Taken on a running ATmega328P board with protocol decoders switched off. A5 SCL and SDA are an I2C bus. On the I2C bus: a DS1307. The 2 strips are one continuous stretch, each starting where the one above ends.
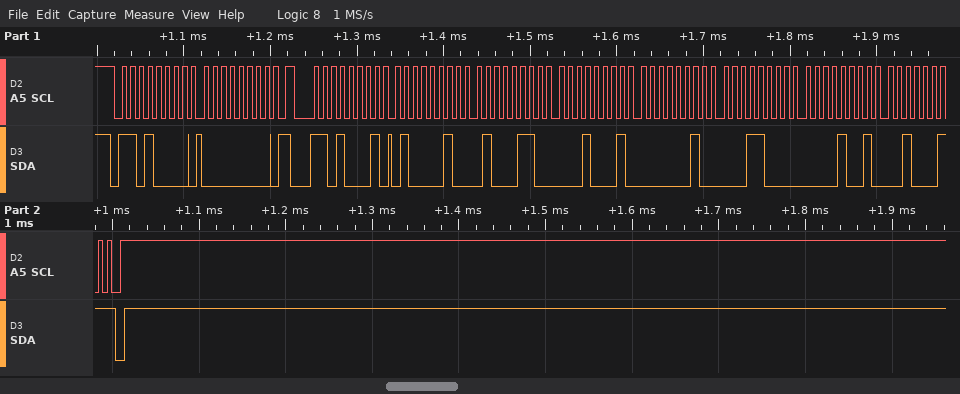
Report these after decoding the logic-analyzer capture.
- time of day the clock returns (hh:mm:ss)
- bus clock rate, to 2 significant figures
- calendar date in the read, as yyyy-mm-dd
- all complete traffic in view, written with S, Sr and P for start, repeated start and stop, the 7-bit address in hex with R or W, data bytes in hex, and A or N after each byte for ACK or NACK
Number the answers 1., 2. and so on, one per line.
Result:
1. 11:46:42
2. 100 kHz
3. 2023-09-18
4. S 68W A 00 A Sr 68R A 42 A 46 A 11 A 02 A 18 A 09 A 23 N P
